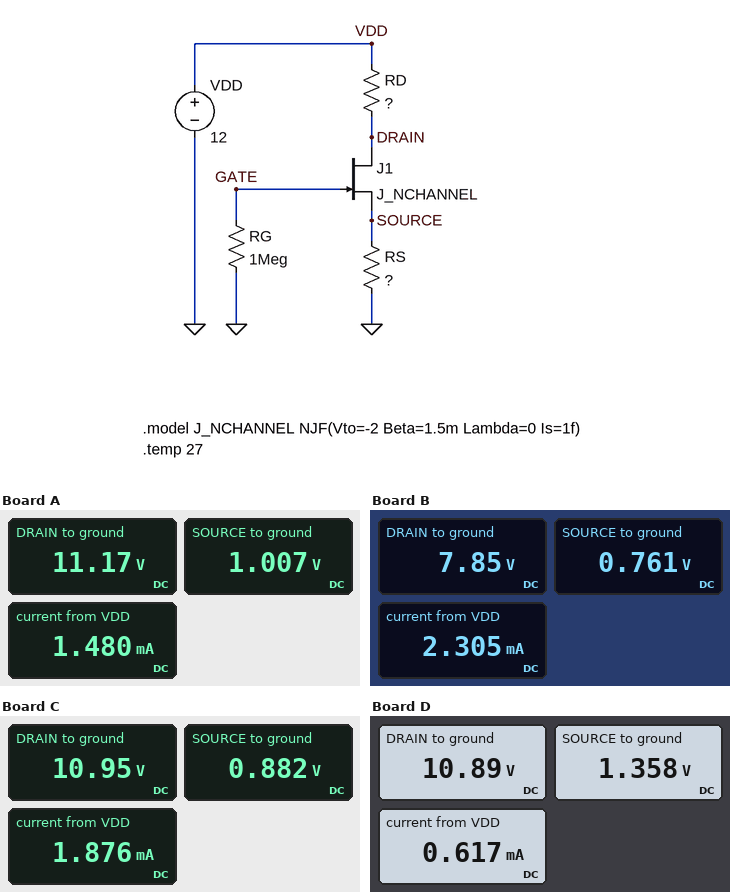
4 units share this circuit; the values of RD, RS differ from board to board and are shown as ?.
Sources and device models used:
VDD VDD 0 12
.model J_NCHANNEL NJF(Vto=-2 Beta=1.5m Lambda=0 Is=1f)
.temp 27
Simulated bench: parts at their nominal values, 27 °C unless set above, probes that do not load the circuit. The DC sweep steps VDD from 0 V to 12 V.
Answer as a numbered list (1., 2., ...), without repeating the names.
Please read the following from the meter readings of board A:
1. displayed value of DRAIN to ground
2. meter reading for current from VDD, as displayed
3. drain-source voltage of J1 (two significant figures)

1. 11.17 V
2. 1.480 mA
3. 10 V
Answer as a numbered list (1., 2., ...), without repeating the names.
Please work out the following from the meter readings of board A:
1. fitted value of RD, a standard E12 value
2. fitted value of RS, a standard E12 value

1. 560 Ω
2. 680 Ω
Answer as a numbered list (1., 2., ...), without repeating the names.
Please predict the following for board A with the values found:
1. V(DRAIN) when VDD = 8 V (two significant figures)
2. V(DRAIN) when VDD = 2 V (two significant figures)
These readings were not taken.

1. 7.2 V
2. 1.3 V
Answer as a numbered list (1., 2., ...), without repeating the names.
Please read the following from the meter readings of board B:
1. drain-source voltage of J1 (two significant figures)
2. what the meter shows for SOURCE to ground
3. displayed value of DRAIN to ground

1. 7.1 V
2. 0.761 V
3. 7.85 V
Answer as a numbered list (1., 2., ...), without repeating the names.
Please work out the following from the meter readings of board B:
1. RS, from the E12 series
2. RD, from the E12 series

1. 330 Ω
2. 1.8 kΩ
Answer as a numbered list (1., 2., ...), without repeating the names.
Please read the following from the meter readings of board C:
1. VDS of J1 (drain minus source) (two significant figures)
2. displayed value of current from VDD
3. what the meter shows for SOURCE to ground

1. 10 V
2. 1.876 mA
3. 0.882 V
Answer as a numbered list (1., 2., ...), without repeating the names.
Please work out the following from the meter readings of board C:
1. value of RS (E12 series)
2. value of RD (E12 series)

1. 470 Ω
2. 560 Ω
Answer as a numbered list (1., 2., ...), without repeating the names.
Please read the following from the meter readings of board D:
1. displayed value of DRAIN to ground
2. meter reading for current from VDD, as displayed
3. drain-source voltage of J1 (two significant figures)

1. 10.89 V
2. 0.617 mA
3. 9.5 V
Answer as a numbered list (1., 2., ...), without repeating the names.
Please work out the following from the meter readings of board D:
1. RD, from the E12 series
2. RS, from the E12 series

1. 1.8 kΩ
2. 2.2 kΩ
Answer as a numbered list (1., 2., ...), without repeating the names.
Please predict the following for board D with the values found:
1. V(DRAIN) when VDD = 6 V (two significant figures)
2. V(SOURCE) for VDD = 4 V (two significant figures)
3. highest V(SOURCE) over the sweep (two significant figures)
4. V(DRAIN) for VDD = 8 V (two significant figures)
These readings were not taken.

1. 4.9 V
2. 1.4 V
3. 1.4 V
4. 6.9 V
